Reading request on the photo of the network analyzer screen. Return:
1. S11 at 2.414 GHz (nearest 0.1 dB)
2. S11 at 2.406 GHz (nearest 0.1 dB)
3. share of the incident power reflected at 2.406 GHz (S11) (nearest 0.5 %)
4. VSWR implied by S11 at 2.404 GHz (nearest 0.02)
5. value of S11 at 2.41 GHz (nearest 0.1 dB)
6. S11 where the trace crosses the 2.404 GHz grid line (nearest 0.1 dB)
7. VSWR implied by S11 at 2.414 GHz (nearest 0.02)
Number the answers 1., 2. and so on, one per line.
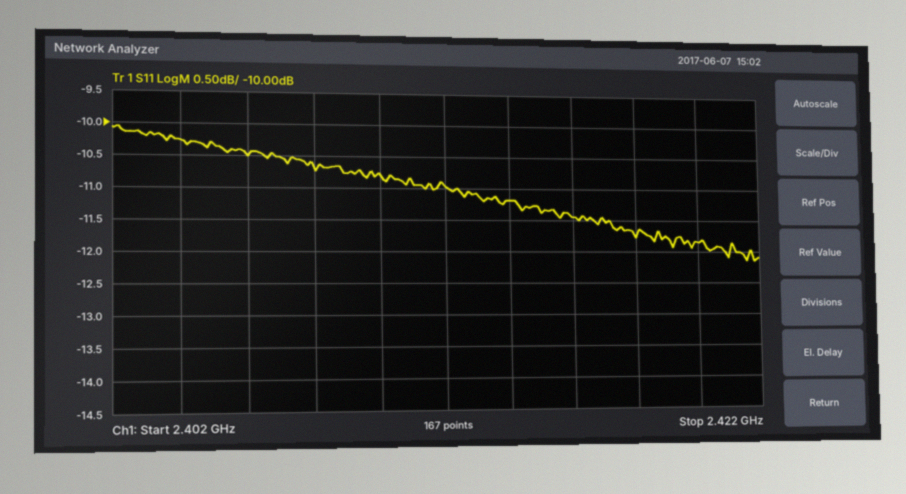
1. -11.2 dB
2. -10.5 dB
3. 9.0 %
4. 1.88
5. -10.8 dB
6. -10.3 dB
7. 1.76
